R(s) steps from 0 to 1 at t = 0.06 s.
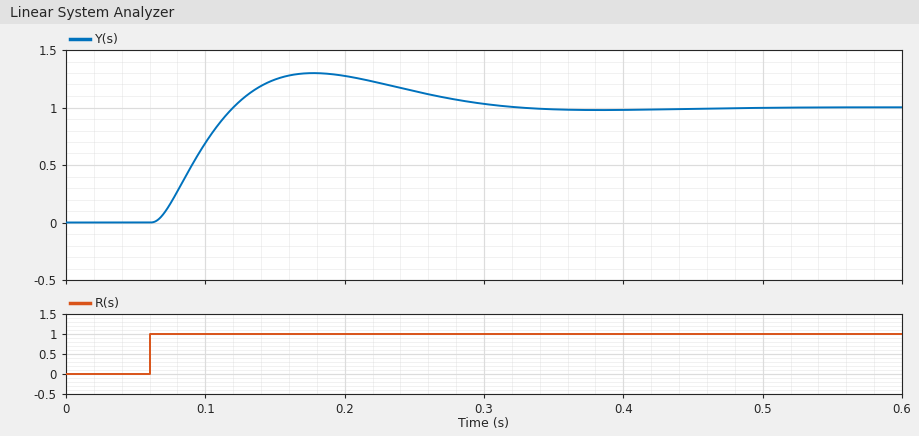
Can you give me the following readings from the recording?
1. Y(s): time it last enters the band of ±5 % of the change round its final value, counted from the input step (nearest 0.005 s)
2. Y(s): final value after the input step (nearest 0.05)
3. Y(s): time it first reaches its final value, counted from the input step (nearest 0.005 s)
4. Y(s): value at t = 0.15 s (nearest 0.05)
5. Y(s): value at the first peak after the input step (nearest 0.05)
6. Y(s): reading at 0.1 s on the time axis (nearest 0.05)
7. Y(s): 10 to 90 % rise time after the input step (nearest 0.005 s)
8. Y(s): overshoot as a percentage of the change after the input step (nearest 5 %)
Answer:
0.230 s
1.00
0.060 s
1.25
1.30
0.70
0.040 s
30 %
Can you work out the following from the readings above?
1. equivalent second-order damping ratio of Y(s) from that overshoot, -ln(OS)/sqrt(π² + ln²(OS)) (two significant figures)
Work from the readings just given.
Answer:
0.36
